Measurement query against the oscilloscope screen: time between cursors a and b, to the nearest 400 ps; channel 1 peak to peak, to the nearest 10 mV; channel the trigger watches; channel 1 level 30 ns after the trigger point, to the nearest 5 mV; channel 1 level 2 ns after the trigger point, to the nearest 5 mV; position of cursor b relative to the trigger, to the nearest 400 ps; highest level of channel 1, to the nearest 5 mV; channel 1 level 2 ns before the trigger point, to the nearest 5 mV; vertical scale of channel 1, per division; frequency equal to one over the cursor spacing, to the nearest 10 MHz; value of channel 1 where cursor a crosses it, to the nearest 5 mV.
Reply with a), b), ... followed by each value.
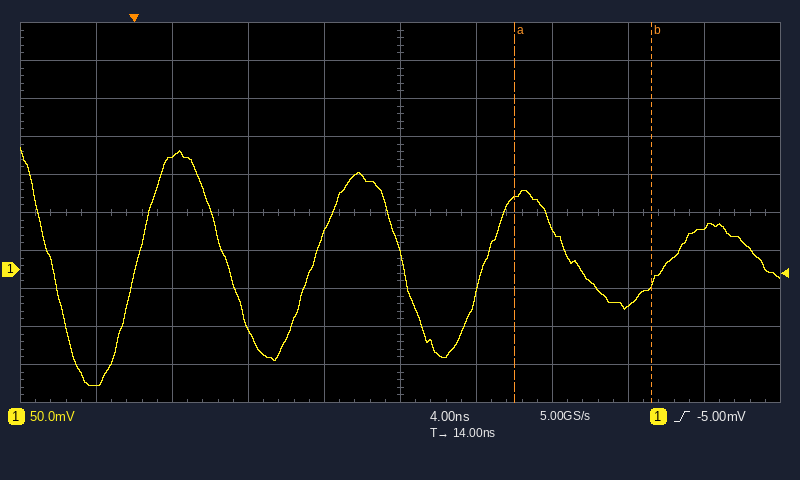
a) 7.2 ns
b) 310 mV
c) channel 1
d) 55 mV
e) 150 mV
f) +27.2 ns
g) 160 mV
h) -150 mV
i) 50 mV
j) 140 MHz
k) 95 mV
